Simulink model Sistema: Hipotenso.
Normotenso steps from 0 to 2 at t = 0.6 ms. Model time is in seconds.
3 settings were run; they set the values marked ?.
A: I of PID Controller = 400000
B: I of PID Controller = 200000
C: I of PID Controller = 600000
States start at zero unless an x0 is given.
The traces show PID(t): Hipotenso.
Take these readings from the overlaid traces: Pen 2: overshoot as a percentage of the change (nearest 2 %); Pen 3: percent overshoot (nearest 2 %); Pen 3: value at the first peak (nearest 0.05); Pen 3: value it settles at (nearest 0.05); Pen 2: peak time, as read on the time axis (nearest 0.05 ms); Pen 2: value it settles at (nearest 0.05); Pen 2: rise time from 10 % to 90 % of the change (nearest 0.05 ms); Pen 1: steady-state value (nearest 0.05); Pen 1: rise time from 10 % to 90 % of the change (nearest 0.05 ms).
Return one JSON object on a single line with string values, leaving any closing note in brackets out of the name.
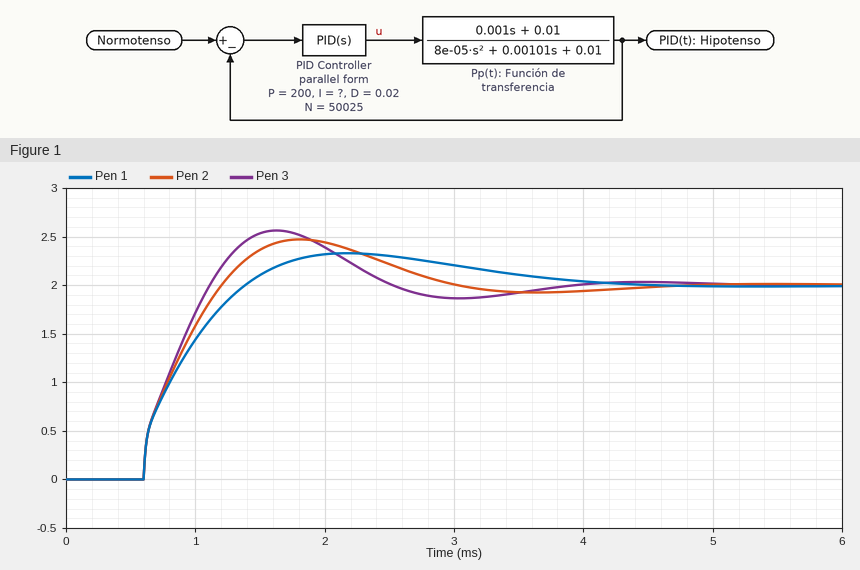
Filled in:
{"Pen 2: overshoot as a percentage of the change": "24 %", "Pen 3: percent overshoot": "28 %", "Pen 3: value at the first peak": "2.55", "Pen 3: value it settles at": "2.00", "Pen 2: peak time, as read on the time axis": "1.80 ms", "Pen 2: value it settles at": "2.00", "Pen 2: rise time from 10 % to 90 % of the change": "0.50 ms", "Pen 1: steady-state value": "2.00", "Pen 1: rise time from 10 % to 90 % of the change": "0.60 ms"}
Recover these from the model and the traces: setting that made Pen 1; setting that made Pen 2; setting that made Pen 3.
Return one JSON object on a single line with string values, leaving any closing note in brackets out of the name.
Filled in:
{"setting that made Pen 1": "B", "setting that made Pen 2": "A", "setting that made Pen 3": "C"}
